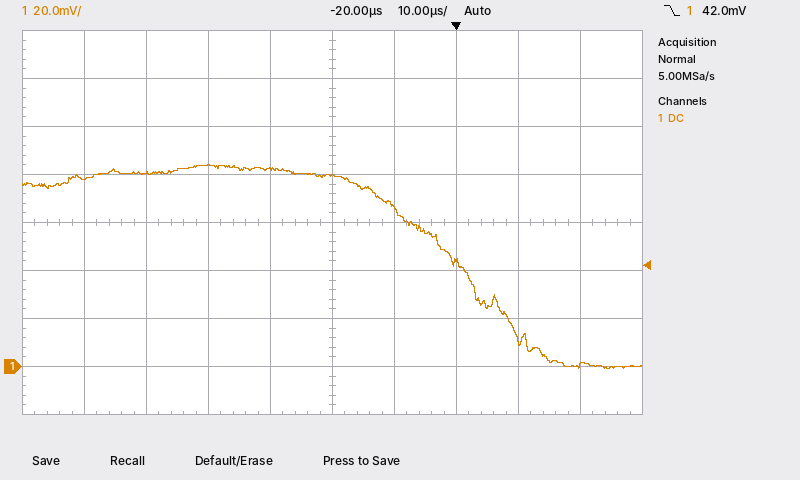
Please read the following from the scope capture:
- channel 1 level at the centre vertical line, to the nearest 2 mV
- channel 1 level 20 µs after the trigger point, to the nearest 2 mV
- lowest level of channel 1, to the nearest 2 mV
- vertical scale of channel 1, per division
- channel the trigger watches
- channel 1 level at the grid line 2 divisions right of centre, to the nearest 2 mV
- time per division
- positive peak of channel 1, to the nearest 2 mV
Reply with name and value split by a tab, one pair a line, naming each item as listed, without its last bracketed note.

channel 1 level at the centre vertical line, to the nearest 2 mV	80 mV
channel 1 level 20 µs after the trigger point, to the nearest 2 mV	0 mV
lowest level of channel 1, to the nearest 2 mV	0 mV
vertical scale of channel 1, per division	20 mV
channel the trigger watches	channel 1
channel 1 level at the grid line 2 divisions right of centre, to the nearest 2 mV	44 mV
time per division	10 µs
positive peak of channel 1, to the nearest 2 mV	84 mV
